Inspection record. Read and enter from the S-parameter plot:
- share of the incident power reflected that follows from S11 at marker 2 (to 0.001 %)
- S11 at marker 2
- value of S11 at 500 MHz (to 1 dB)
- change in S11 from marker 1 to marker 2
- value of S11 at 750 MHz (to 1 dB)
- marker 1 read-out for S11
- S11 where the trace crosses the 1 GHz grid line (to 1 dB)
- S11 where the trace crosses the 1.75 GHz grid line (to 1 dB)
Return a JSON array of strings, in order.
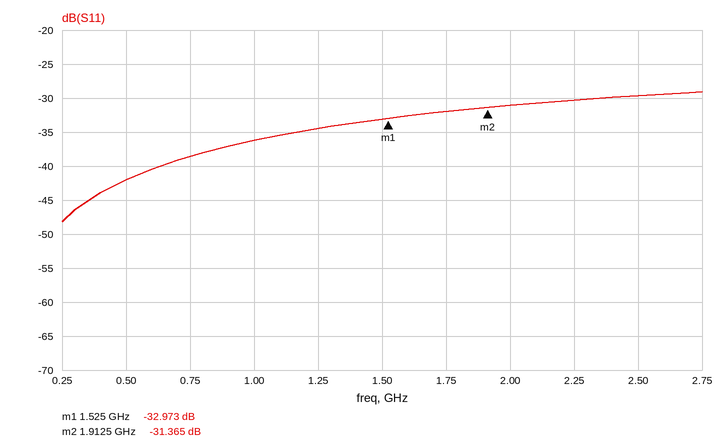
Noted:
["0.073 %", "-31.365 dB", "-42 dB", "1.608 dB", "-39 dB", "-32.973 dB", "-36 dB", "-32 dB"]
